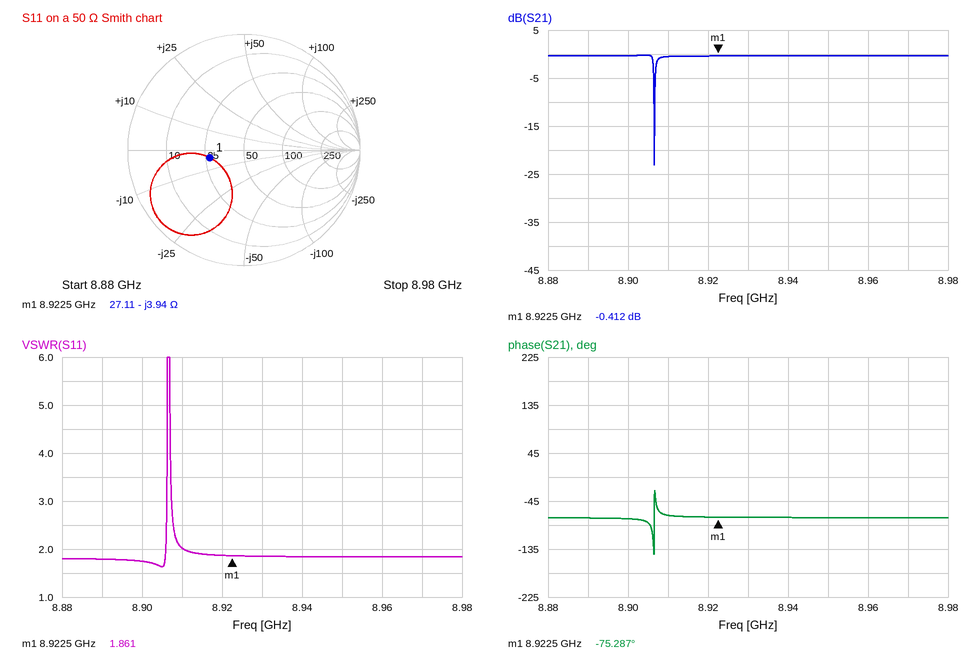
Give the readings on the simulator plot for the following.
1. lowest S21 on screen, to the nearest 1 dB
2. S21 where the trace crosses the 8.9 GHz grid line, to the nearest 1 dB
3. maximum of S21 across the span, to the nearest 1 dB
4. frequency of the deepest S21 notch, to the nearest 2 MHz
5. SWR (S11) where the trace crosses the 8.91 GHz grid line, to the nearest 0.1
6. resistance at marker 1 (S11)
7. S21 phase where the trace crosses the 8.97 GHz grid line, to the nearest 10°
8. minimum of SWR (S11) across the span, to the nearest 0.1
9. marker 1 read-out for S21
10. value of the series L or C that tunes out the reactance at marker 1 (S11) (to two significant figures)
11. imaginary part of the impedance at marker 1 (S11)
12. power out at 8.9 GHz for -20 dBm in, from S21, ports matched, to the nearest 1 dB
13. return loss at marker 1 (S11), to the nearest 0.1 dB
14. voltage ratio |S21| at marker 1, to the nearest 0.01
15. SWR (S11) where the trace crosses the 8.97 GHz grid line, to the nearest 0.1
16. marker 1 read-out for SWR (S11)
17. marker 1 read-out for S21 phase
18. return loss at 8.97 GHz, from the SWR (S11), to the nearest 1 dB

-23 dB
0 dB
0 dB
8.906 GHz
2.0
27.11 Ω
-80°
1.6
-0.412 dB
70 pH
-3.94 Ω
-20 dBm
10.4 dB
0.95
1.8
1.861
-75.287°
11 dB
